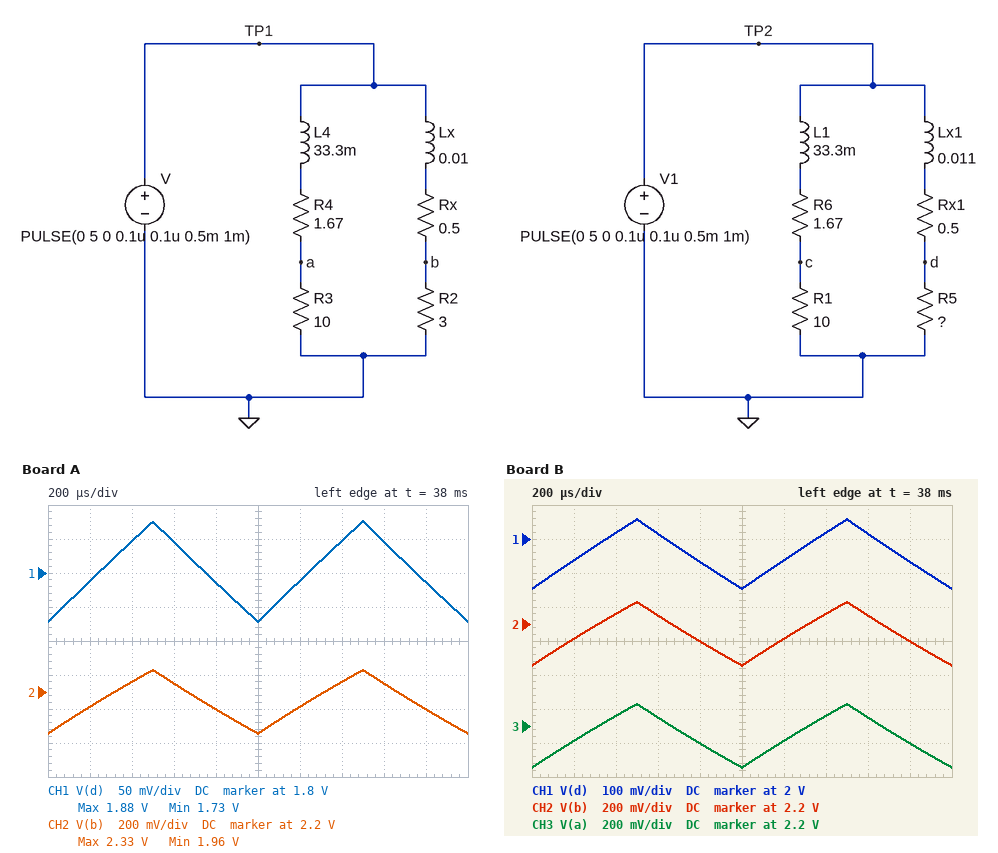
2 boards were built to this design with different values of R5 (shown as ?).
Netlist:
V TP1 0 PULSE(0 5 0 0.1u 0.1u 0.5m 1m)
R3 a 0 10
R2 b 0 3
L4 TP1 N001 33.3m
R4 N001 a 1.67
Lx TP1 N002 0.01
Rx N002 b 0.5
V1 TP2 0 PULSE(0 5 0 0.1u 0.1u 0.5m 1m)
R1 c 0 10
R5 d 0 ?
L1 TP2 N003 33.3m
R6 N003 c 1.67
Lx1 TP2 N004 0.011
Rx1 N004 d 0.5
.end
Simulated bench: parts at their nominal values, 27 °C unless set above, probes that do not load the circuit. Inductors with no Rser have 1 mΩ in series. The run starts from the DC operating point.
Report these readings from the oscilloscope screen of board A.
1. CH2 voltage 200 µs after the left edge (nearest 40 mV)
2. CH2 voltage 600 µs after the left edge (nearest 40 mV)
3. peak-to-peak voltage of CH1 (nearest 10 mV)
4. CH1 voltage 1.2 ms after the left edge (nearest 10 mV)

2.12 V
2.24 V
150 mV
1.79 V
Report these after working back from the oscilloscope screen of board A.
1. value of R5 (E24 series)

1.3 Ω
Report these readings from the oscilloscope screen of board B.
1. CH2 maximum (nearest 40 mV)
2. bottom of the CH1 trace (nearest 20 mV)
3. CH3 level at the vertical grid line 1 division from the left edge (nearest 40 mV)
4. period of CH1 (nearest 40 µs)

2.32 V
1.86 V
2.12 V
1.00 ms
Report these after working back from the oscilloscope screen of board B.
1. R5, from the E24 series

1.8 Ω
